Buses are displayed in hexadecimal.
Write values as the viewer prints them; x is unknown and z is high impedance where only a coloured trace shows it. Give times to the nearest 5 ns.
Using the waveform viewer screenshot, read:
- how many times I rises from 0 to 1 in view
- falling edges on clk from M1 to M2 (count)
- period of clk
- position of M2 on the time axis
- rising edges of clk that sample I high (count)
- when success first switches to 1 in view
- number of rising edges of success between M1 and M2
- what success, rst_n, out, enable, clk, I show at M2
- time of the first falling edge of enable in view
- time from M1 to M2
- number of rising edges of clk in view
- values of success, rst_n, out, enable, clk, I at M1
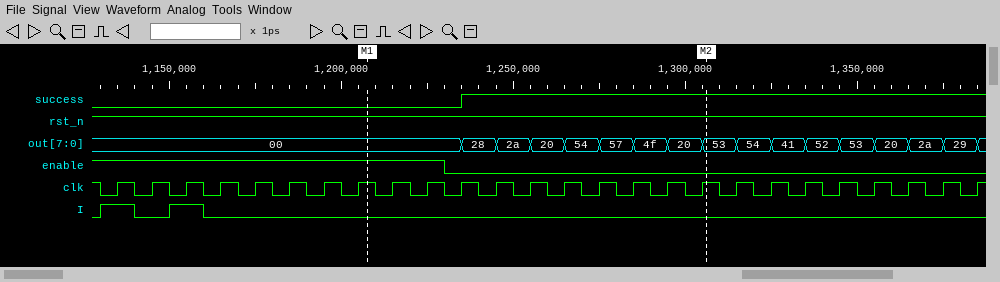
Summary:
2
10
10 ns
1305 ns
2
1235 ns
1
success=1, rst_n=1, out=53, enable=0, clk=1, I=0
1230 ns
100 ns
26
success=0, rst_n=1, out=00, enable=1, clk=1, I=0
